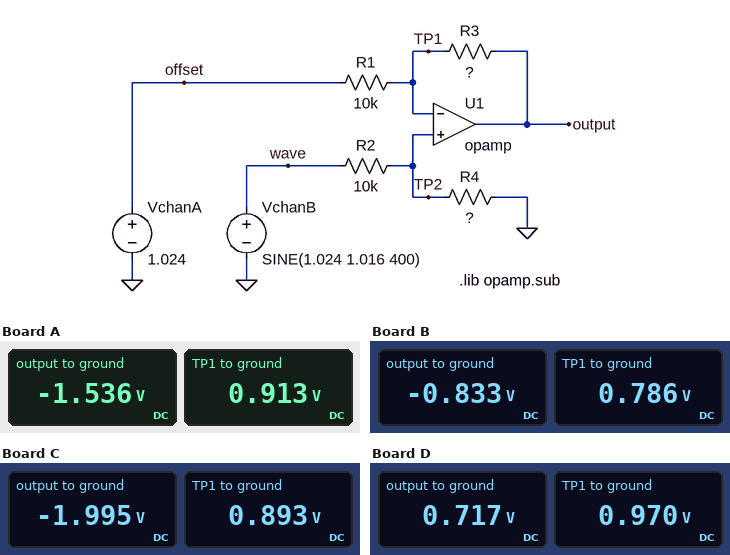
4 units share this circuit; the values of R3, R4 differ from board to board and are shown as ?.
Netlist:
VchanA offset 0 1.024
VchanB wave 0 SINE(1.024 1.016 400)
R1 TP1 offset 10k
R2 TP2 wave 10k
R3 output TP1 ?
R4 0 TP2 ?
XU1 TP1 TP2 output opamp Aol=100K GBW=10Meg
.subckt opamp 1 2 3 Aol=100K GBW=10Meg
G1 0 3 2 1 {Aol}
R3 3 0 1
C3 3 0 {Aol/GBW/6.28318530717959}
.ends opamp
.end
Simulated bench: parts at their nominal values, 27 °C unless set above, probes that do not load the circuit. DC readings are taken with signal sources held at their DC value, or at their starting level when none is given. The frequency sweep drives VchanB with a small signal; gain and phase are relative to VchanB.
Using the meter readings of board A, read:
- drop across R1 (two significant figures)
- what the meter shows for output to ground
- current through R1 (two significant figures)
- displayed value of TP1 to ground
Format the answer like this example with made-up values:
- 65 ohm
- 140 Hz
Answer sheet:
- 110 mV
- -1.536 V
- 11 µA
- 0.913 V
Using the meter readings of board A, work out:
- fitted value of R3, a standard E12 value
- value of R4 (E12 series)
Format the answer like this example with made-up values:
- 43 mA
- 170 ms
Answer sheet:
- 220 kΩ
- 82 kΩ
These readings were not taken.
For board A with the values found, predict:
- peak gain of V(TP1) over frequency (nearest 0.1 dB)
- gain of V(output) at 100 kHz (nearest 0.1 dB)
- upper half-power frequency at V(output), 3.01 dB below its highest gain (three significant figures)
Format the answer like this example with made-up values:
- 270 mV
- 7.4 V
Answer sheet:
- -1.0 dB
- 26.0 dB
- 435 kHz
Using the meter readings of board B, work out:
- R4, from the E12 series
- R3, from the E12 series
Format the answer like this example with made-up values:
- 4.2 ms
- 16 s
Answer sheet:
- 33 kΩ
- 68 kΩ
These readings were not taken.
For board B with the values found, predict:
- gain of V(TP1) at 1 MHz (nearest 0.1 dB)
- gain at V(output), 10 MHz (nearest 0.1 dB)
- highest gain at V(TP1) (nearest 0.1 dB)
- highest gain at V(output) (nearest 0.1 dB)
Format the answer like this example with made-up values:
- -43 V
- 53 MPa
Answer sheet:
- -4.4 dB
- -2.4 dB
- -2.3 dB
- 15.5 dB
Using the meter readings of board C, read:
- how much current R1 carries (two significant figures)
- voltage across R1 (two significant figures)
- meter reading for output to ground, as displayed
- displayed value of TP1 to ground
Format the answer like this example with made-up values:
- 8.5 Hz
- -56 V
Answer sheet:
- 13 µA
- 130 mV
- -1.995 V
- 0.893 V
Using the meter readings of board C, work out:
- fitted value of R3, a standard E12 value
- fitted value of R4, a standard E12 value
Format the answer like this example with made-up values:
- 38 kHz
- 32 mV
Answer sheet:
- 220 kΩ
- 68 kΩ
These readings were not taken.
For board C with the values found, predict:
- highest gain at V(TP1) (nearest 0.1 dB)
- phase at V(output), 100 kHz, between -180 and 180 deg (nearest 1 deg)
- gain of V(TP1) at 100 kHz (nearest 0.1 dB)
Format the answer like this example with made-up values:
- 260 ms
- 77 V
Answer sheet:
- -1.2 dB
- -13 deg
- -1.4 dB
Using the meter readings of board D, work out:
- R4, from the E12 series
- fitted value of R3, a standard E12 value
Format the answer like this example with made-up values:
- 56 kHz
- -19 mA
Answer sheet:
- 180 kΩ
- 47 kΩ
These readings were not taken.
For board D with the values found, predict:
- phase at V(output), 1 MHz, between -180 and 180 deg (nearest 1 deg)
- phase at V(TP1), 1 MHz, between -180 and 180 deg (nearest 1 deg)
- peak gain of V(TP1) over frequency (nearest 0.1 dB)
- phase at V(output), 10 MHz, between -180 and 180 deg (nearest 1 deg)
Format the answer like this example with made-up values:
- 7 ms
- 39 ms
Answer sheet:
- -30 deg
- -30 deg
- -0.5 dB
- -80 deg
